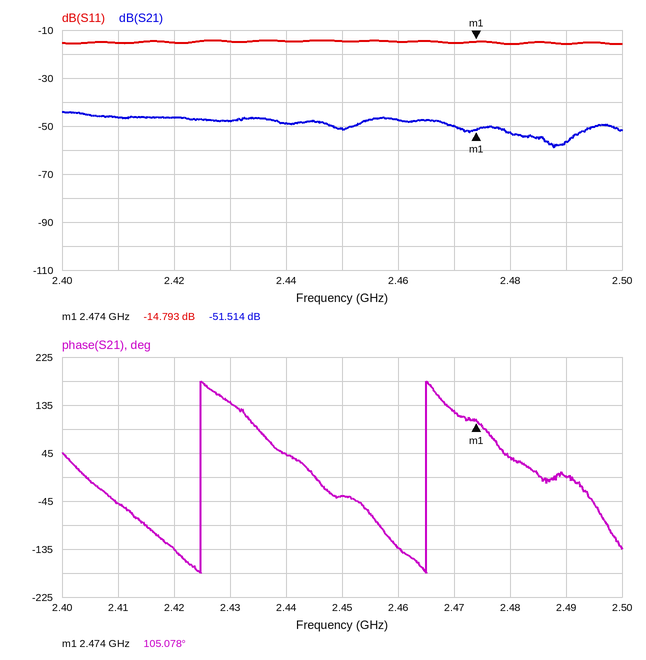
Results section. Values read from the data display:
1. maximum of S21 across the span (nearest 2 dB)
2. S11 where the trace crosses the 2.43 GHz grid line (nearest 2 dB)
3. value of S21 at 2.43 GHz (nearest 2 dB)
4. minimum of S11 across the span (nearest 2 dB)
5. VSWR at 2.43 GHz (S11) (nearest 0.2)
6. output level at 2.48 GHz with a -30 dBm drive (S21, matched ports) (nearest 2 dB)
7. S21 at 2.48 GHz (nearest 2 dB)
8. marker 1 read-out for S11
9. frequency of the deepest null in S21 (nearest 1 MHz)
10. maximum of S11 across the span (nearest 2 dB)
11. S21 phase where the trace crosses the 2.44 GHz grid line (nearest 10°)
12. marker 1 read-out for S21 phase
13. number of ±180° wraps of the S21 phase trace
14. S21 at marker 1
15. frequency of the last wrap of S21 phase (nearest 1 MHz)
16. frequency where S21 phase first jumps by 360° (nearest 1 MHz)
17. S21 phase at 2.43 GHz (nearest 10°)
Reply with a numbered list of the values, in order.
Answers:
1. -44 dB
2. -14 dB
3. -48 dB
4. -16 dB
5. 1.4
6. -82 dBm
7. -52 dB
8. -14.793 dB
9. 2.488 GHz
10. -14 dB
11. 40°
12. 105.078°
13. 2
14. -51.514 dB
15. 2.465 GHz
16. 2.425 GHz
17. 140°
